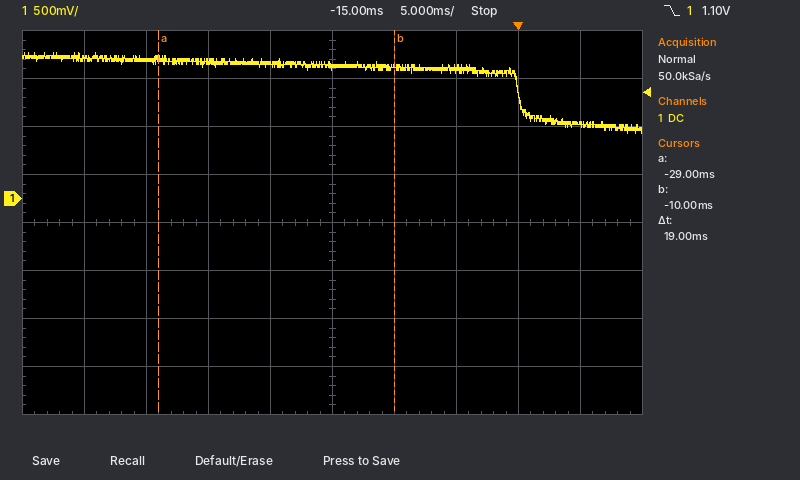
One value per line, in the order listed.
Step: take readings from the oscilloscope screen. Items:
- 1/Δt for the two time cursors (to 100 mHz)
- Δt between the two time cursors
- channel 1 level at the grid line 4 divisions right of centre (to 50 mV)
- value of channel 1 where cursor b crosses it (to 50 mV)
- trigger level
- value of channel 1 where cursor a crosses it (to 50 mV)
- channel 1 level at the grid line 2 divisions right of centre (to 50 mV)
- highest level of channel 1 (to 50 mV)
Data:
52.6 Hz
19 ms
750 mV
1.35 V
1.10 V
1.45 V
1.35 V
1.50 V
